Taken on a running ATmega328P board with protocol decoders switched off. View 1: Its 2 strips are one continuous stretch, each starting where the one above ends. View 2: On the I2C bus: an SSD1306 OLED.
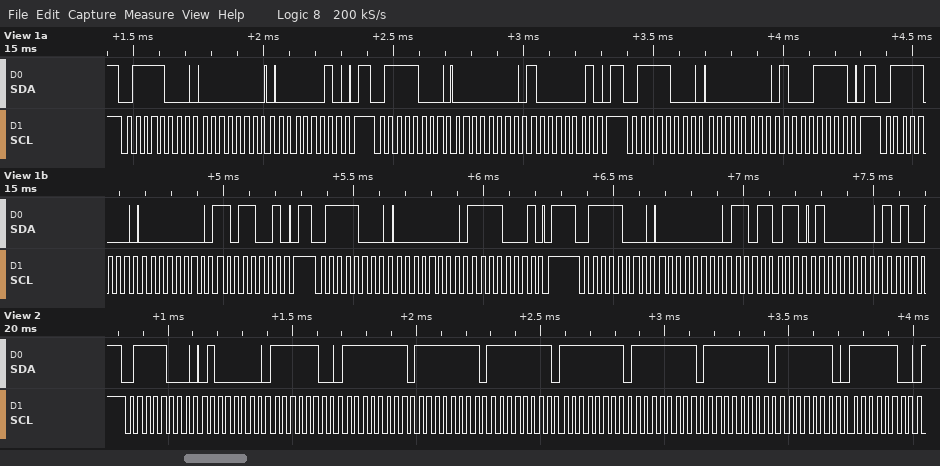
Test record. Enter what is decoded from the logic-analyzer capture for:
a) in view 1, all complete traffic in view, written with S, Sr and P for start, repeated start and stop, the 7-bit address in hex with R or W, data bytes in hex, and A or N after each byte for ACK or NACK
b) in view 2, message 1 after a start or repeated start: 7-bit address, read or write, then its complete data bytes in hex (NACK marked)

S 3CW A 00 A 02 A P S 3CW A 00 A 81 A P S 3CW A 00 A 8F A P S 3CW A 00 A D9 A P S 3CW A 00 A F1 A P S 3CW A 00 A DB A 40 A
0x3C write: 40 FC FF FF FF FF FF FF FE FC
